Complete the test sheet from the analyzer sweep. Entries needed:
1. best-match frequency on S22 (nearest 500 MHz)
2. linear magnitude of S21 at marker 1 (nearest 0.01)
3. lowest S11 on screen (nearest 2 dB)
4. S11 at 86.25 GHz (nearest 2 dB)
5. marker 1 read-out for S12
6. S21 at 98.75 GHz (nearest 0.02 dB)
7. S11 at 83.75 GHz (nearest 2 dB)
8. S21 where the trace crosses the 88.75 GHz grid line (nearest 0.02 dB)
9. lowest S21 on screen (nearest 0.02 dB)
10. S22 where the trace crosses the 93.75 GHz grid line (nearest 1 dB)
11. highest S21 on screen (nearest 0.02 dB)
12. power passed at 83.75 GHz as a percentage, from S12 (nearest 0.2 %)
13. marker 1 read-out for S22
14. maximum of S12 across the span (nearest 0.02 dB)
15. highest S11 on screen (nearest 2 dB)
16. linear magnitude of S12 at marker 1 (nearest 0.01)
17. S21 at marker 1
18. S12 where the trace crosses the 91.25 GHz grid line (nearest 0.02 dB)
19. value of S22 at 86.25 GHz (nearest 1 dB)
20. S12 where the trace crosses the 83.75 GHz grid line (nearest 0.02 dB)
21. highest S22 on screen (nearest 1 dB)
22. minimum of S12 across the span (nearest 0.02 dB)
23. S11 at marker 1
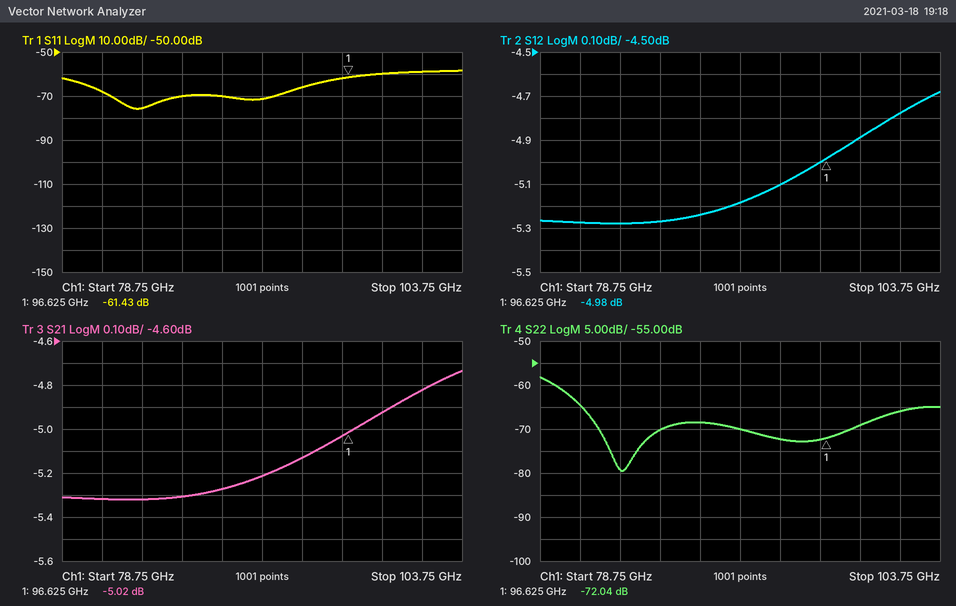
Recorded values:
84.0 GHz
0.56
-76 dB
-70 dB
-4.98 dB
-4.92 dB
-76 dB
-5.28 dB
-5.32 dB
-72 dB
-4.74 dB
29.6 %
-72.04 dB
-4.68 dB
-58 dB
0.56
-5.02 dB
-5.18 dB
-70 dB
-5.28 dB
-58 dB
-5.28 dB
-61.43 dB
